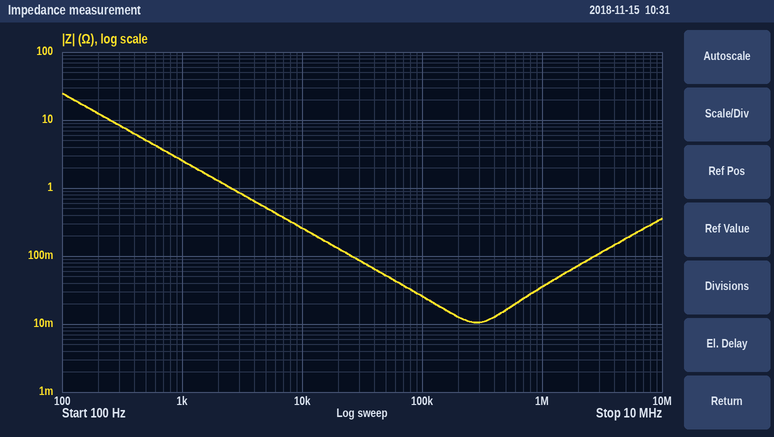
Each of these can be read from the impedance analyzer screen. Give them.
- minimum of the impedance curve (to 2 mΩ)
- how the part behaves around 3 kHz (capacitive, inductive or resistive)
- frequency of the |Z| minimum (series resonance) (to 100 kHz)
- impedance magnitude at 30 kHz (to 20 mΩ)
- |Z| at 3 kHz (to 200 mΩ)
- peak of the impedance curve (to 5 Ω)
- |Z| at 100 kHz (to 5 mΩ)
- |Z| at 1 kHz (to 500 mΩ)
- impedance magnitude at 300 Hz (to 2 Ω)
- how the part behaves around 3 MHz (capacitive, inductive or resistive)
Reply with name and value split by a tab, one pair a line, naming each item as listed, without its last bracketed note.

minimum of the impedance curve	10 mΩ
how the part behaves around 3 kHz	capacitive
frequency of the |Z| minimum (series resonance)	300 kHz
impedance magnitude at 30 kHz	80 mΩ
|Z| at 3 kHz	800 mΩ
peak of the impedance curve	25 Ω
|Z| at 100 kHz	25 mΩ
|Z| at 1 kHz	2.5 Ω
impedance magnitude at 300 Hz	8 Ω
how the part behaves around 3 MHz	inductive
